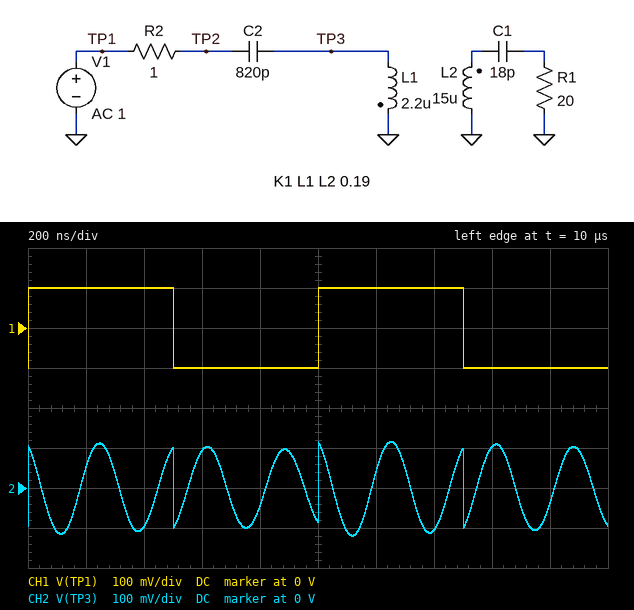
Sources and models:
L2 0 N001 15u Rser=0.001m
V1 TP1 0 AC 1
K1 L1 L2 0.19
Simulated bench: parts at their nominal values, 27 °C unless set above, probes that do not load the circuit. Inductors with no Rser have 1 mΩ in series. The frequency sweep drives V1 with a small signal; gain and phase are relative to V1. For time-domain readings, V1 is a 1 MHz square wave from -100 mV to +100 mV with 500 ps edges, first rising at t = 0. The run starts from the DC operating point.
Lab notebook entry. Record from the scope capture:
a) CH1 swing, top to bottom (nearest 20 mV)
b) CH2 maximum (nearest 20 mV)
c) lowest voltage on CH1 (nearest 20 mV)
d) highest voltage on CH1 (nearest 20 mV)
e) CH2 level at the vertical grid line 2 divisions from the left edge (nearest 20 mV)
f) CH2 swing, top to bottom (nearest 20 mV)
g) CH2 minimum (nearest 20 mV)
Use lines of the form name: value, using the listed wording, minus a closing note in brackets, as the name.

CH1 swing, top to bottom: 200 mV
CH2 maximum: 120 mV
lowest voltage on CH1: -100 mV
highest voltage on CH1: 100 mV
CH2 level at the vertical grid line 2 divisions from the left edge: -100 mV
CH2 swing, top to bottom: 240 mV
CH2 minimum: -120 mV
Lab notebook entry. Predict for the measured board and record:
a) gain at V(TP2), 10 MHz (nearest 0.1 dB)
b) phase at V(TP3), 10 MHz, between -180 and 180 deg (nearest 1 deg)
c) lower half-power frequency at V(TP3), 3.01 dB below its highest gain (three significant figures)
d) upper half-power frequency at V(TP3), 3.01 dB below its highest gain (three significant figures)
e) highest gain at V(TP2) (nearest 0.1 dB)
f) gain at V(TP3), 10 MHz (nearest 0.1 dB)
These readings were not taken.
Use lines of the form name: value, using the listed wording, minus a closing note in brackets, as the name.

gain at V(TP2), 10 MHz: -0.1 dB
phase at V(TP3), 10 MHz, between -180 and 180 deg: 8 deg
lower half-power frequency at V(TP3), 3.01 dB below its highest gain: 3.70 MHz
upper half-power frequency at V(TP3), 3.01 dB below its highest gain: 3.77 MHz
highest gain at V(TP2): 0 dB
gain at V(TP3), 10 MHz: 2.4 dB
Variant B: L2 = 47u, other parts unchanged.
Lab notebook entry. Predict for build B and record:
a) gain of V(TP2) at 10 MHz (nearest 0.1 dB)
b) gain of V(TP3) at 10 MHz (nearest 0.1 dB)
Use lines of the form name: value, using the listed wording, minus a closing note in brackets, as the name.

gain of V(TP2) at 10 MHz: 0 dB
gain of V(TP3) at 10 MHz: 1.4 dB
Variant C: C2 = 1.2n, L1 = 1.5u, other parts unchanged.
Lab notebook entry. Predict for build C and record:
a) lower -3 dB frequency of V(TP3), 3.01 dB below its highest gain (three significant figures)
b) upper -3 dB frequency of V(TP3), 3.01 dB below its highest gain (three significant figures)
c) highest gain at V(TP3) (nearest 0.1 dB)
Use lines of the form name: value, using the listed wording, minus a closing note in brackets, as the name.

lower -3 dB frequency of V(TP3), 3.01 dB below its highest gain: 3.69 MHz
upper -3 dB frequency of V(TP3), 3.01 dB below its highest gain: 3.79 MHz
highest gain at V(TP3): 31.0 dB
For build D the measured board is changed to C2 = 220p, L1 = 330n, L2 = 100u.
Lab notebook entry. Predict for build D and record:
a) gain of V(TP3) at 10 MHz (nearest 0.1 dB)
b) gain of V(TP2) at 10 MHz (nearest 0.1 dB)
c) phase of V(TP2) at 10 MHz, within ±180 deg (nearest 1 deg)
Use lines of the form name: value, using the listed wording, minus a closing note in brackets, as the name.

gain of V(TP3) at 10 MHz: -8.4 dB
gain of V(TP2) at 10 MHz: 0 dB
phase of V(TP2) at 10 MHz, within ±180 deg: -1 deg
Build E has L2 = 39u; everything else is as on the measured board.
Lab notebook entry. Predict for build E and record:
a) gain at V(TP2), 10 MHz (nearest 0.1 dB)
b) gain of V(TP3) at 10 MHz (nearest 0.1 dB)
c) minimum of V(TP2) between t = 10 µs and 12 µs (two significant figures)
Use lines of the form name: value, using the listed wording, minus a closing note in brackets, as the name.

gain at V(TP2), 10 MHz: 0 dB
gain of V(TP3) at 10 MHz: 1.4 dB
minimum of V(TP2) between t = 10 µs and 12 µs: -100 mV
